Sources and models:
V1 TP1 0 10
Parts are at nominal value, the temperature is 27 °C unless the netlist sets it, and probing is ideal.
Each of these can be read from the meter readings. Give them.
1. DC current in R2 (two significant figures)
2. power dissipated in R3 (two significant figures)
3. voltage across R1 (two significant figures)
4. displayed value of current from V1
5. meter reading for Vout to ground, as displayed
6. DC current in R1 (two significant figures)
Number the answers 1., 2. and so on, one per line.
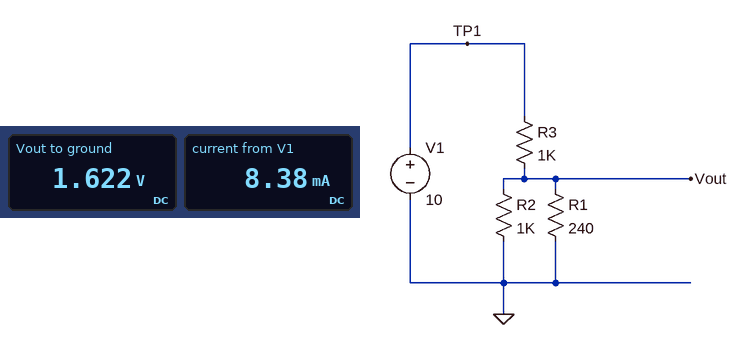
1. 1.6 mA
2. 70 mW
3. 1.6 V
4. 8.38 mA
5. 1.622 V
6. 6.8 mA
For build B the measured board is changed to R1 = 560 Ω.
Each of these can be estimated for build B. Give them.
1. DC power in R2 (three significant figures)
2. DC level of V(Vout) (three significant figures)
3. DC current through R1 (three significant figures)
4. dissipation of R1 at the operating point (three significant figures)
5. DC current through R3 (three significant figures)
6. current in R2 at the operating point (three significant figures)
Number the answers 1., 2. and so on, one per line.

1. 6.98 mW
2. 2.64 V
3. 4.72 mA
4. 12.5 mW
5. 7.36 mA
6. 2.64 mA
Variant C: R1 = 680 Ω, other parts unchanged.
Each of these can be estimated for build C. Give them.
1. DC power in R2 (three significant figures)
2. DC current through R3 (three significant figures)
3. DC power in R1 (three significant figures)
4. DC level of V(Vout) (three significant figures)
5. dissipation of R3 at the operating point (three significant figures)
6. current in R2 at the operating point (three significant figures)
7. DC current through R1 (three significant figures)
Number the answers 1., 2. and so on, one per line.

1. 8.30 mW
2. 7.12 mA
3. 12.2 mW
4. 2.88 V
5. 50.7 mW
6. 2.88 mA
7. 4.24 mA
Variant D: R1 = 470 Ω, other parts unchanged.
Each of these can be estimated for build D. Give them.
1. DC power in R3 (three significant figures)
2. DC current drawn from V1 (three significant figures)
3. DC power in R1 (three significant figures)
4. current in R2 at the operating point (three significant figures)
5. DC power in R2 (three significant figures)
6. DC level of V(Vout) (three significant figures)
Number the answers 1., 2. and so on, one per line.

1. 57.4 mW
2. 7.58 mA
3. 12.5 mW
4. 2.42 mA
5. 5.87 mW
6. 2.42 V
